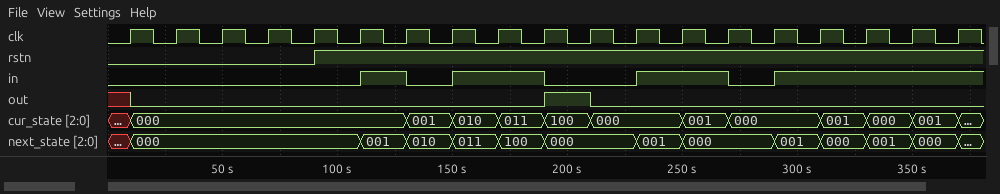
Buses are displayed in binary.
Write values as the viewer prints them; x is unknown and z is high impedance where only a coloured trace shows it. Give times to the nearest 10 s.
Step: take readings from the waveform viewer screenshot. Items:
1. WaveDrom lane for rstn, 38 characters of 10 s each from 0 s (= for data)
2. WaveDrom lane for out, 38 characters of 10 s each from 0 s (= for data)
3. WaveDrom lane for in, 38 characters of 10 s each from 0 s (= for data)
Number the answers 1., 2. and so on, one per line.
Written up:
1. {name: 'rstn', wave: '0........1............................'}
2. {name: 'out', wave: 'x0.................1.0................'}
3. {name: 'in', wave: '0..........1.0.1...0...1...0.1........'}
